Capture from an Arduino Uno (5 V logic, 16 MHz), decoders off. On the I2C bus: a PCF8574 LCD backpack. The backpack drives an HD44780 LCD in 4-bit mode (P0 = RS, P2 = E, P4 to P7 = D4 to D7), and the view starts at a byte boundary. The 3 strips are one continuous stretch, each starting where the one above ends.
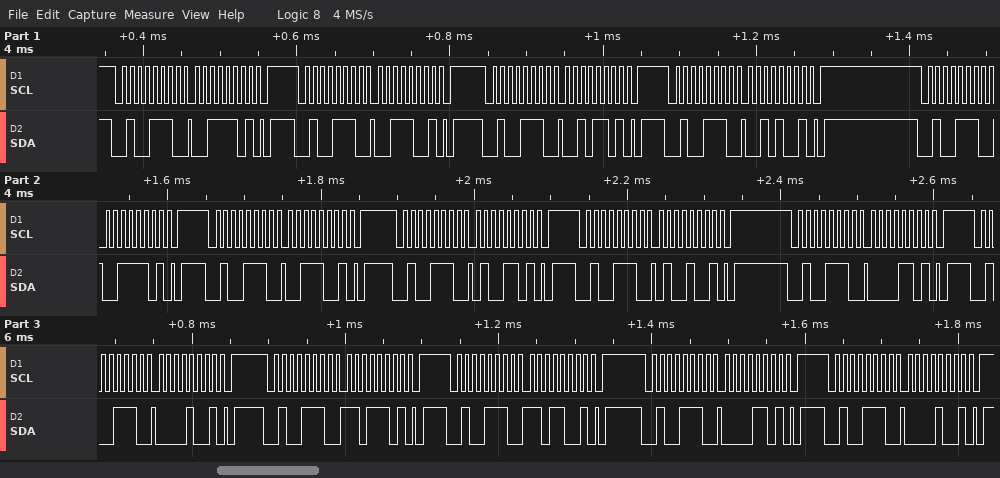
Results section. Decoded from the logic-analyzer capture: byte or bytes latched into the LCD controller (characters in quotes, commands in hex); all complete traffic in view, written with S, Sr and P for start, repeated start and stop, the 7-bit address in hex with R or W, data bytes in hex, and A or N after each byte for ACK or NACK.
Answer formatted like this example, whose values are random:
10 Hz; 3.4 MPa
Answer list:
'2' '4' data 0x0D; S 27W A 3D A P S 27W A 39 A P S 27W A 2D A P S 27W A 29 A P S 27W A 3D A P S 27W A 39 A P S 27W A 4D A P S 27W A 49 A P S 27W A 0D A P S 27W A 09 A P S 27W A DD A P S 27W A D9 A P S 27W A 0D A P S 27W A 09 A P
